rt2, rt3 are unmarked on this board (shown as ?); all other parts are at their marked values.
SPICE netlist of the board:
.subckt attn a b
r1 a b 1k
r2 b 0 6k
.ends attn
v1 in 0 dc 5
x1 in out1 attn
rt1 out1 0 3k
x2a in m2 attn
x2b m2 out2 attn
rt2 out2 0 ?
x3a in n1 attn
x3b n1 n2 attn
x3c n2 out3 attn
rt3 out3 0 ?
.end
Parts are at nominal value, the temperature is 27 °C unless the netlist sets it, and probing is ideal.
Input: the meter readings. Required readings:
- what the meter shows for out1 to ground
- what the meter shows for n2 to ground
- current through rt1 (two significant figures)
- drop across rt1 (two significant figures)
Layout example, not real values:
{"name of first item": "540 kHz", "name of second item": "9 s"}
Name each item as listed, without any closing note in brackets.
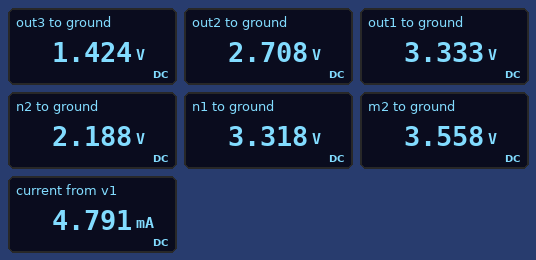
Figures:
{"what the meter shows for out1 to ground": "3.333 V", "what the meter shows for n2 to ground": "2.188 V", "current through rt1": "1.1 mA", "drop across rt1": "3.3 V"}
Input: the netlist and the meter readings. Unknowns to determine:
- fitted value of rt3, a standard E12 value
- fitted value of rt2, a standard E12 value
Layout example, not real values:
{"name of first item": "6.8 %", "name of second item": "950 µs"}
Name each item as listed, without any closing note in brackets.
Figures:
{"fitted value of rt3, a standard E12 value": "2.7 kΩ", "fitted value of rt2, a standard E12 value": "6.8 kΩ"}
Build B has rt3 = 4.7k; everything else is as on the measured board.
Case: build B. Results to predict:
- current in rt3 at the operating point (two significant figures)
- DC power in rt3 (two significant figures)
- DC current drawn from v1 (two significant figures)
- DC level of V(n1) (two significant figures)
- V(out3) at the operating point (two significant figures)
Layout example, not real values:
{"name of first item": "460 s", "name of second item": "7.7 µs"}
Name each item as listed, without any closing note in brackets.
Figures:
{"current in rt3 at the operating point": "360 µA", "DC power in rt3": "620 µW", "DC current drawn from v1": "4.7 mA", "DC level of V(n1)": "3.4 V", "V(out3) at the operating point": "1.7 V"}
